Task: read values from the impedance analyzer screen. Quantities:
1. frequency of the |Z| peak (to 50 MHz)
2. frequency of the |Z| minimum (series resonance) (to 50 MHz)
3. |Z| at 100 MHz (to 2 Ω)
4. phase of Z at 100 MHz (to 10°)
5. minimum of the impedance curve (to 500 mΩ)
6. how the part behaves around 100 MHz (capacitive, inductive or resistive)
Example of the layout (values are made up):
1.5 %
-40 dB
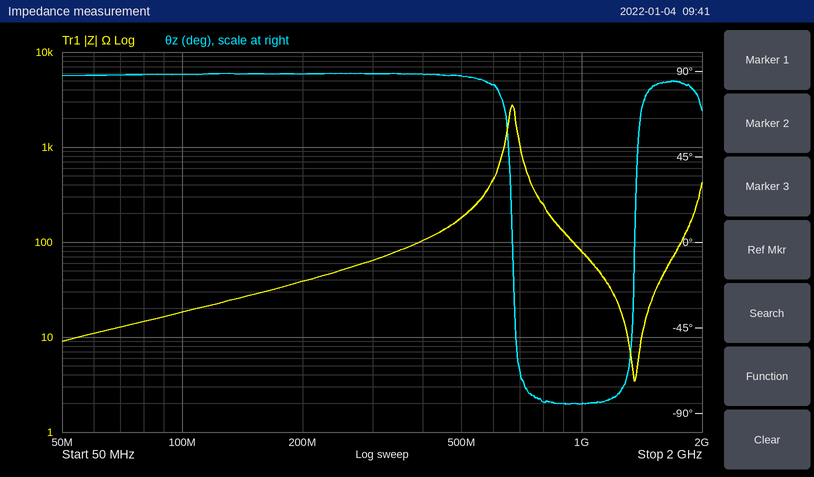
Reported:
650 MHz
1.35 GHz
18 Ω
90°
3.5 Ω
inductive
